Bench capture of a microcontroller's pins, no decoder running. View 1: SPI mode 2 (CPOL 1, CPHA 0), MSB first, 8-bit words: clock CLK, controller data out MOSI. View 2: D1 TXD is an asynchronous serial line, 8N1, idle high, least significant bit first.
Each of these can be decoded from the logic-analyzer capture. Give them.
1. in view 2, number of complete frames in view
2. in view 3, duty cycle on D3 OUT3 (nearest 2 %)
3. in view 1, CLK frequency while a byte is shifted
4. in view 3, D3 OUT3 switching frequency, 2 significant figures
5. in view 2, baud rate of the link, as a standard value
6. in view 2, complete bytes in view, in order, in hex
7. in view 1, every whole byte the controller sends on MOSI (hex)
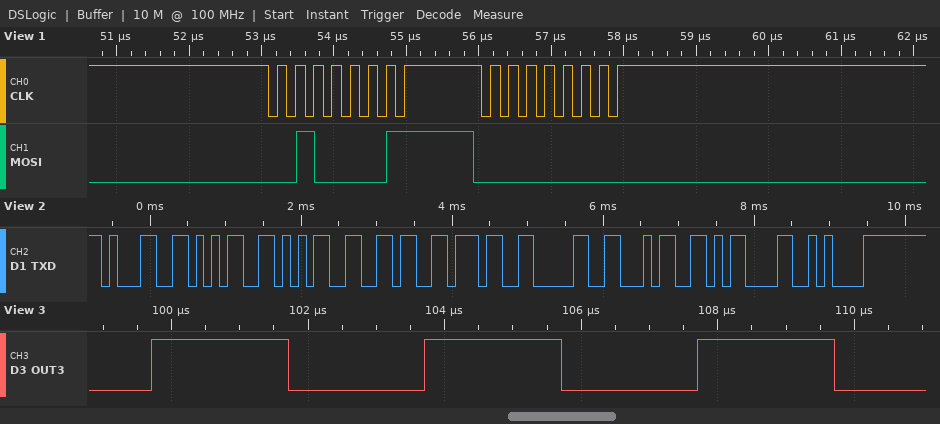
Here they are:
9
50 %
4 MHz
250 kHz
9600 baud
31 35 35 36 37 30 34 0D 0A
0x21 0x00
